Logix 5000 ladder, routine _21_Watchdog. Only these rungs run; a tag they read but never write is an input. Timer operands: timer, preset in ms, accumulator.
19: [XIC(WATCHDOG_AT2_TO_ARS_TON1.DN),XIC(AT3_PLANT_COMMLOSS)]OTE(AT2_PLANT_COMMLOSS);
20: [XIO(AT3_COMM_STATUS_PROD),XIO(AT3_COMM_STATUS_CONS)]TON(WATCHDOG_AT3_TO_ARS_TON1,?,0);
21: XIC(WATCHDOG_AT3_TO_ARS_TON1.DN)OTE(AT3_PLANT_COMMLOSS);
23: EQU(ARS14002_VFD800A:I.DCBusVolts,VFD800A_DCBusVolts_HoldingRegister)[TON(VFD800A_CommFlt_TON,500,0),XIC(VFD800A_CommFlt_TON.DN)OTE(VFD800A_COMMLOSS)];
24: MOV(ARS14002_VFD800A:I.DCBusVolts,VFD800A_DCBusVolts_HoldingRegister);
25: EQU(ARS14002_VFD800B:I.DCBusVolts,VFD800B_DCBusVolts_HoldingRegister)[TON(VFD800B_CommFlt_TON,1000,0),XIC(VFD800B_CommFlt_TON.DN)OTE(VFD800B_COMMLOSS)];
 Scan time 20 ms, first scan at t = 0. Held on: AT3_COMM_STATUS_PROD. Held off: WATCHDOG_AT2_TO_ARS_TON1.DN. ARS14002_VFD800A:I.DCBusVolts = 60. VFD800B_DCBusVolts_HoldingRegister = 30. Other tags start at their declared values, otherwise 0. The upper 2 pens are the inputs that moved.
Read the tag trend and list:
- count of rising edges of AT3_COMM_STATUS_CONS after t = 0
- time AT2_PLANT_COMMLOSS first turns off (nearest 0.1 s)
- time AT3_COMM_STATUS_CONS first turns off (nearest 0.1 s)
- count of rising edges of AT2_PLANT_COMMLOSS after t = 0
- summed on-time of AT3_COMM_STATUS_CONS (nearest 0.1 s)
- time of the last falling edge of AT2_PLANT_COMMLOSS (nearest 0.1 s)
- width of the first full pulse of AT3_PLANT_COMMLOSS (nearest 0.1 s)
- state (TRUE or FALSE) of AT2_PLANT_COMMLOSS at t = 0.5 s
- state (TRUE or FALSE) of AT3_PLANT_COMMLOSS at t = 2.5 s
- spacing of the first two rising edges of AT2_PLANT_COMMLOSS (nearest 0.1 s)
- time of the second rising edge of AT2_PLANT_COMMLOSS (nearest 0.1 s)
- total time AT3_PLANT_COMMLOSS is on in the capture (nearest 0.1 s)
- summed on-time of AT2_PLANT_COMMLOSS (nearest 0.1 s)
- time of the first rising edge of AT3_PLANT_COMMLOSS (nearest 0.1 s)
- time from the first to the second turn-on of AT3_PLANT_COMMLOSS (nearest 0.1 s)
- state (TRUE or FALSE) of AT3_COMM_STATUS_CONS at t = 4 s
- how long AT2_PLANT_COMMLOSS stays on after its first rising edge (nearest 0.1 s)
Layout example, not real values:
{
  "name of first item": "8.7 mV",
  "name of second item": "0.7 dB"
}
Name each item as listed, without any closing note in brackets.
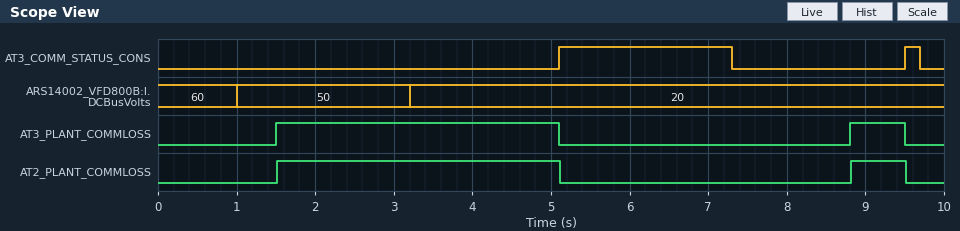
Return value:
{
  "count of rising edges of AT3_COMM_STATUS_CONS after t = 0": "2",
  "time AT2_PLANT_COMMLOSS first turns off": "5.1 s",
  "time AT3_COMM_STATUS_CONS first turns off": "7.3 s",
  "count of rising edges of AT2_PLANT_COMMLOSS after t = 0": "2",
  "summed on-time of AT3_COMM_STATUS_CONS": "2.4 s",
  "time of the last falling edge of AT2_PLANT_COMMLOSS": "9.5 s",
  "width of the first full pulse of AT3_PLANT_COMMLOSS": "3.6 s",
  "state (TRUE or FALSE) of AT2_PLANT_COMMLOSS at t = 0.5 s": "FALSE",
  "state (TRUE or FALSE) of AT3_PLANT_COMMLOSS at t = 2.5 s": "TRUE",
  "spacing of the first two rising edges of AT2_PLANT_COMMLOSS": "7.3 s",
  "time of the second rising edge of AT2_PLANT_COMMLOSS": "8.8 s",
  "total time AT3_PLANT_COMMLOSS is on in the capture": "4.3 s",
  "summed on-time of AT2_PLANT_COMMLOSS": "4.3 s",
  "time of the first rising edge of AT3_PLANT_COMMLOSS": "1.5 s",
  "time from the first to the second turn-on of AT3_PLANT_COMMLOSS": "7.3 s",
  "state (TRUE or FALSE) of AT3_COMM_STATUS_CONS at t = 4 s": "FALSE",
  "how long AT2_PLANT_COMMLOSS stays on after its first rising edge": "3.6 s"
}
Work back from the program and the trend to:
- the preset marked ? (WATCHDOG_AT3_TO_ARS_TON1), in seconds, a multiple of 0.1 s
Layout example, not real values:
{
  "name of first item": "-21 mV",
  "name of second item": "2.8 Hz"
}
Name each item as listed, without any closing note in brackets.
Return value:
{
  "the preset marked ? (WATCHDOG_AT3_TO_ARS_TON1), in seconds, a multiple of 0.1 s": "1.5 s"
}
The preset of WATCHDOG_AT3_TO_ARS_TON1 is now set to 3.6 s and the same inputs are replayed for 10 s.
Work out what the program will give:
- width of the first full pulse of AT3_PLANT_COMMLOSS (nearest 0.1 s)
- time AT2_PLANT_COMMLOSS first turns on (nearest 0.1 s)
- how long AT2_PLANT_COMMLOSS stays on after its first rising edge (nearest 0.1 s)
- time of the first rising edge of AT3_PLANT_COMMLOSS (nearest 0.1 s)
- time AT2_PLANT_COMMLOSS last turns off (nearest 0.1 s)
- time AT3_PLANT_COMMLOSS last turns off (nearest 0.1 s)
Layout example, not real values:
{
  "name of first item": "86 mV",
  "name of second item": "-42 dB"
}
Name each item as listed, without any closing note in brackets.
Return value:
{
  "width of the first full pulse of AT3_PLANT_COMMLOSS": "1.5 s",
  "time AT2_PLANT_COMMLOSS first turns on": "3.6 s",
  "how long AT2_PLANT_COMMLOSS stays on after its first rising edge": "1.5 s",
  "time of the first rising edge of AT3_PLANT_COMMLOSS": "3.6 s",
  "time AT2_PLANT_COMMLOSS last turns off": "5.1 s",
  "time AT3_PLANT_COMMLOSS last turns off": "5.1 s"
}
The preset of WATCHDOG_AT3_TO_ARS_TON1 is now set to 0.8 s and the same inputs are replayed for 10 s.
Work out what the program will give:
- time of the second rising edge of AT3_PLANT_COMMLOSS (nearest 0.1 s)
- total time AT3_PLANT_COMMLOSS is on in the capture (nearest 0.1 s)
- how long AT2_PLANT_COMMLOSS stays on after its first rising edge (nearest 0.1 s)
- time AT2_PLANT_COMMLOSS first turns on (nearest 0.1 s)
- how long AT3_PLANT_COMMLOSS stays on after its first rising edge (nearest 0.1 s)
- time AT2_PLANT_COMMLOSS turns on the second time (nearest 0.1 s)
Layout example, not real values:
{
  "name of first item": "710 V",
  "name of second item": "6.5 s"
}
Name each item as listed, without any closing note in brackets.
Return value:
{
  "time of the second rising edge of AT3_PLANT_COMMLOSS": "8.1 s",
  "total time AT3_PLANT_COMMLOSS is on in the capture": "5.7 s",
  "how long AT2_PLANT_COMMLOSS stays on after its first rising edge": "4.3 s",
  "time AT2_PLANT_COMMLOSS first turns on": "0.8 s",
  "how long AT3_PLANT_COMMLOSS stays on after its first rising edge": "4.3 s",
  "time AT2_PLANT_COMMLOSS turns on the second time": "8.1 s"
}
